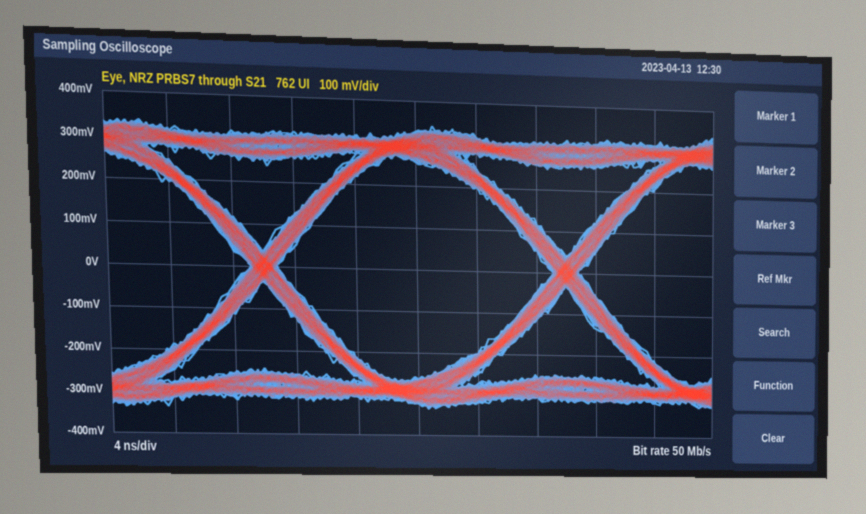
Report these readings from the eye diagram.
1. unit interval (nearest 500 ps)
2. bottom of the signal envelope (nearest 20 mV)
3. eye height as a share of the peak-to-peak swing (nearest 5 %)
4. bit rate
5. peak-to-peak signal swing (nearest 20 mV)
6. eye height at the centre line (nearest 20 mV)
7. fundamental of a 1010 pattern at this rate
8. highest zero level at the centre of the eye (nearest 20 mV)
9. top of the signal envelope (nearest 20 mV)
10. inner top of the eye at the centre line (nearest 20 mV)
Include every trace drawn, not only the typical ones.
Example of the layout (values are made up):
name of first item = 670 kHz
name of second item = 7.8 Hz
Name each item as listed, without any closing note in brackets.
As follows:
unit interval = 20.0 ns
bottom of the signal envelope = -340 mV
eye height as a share of the peak-to-peak swing = 75 %
bit rate = 50 Mb/s
peak-to-peak signal swing = 680 mV
eye height at the centre line = 520 mV
fundamental of a 1010 pattern at this rate = 25 MHz
highest zero level at the centre of the eye = -260 mV
top of the signal envelope = 340 mV
inner top of the eye at the centre line = 260 mV
